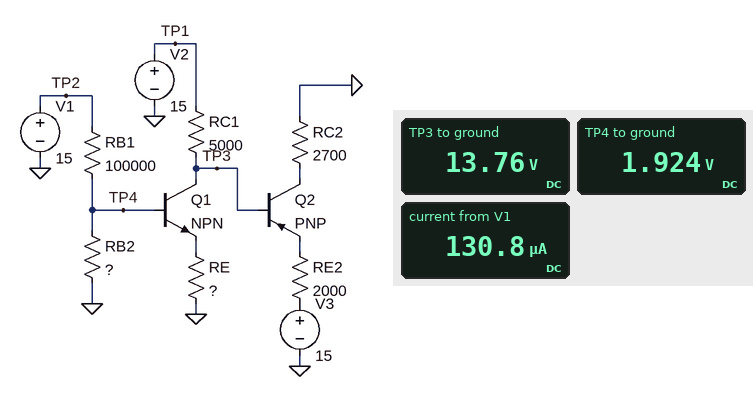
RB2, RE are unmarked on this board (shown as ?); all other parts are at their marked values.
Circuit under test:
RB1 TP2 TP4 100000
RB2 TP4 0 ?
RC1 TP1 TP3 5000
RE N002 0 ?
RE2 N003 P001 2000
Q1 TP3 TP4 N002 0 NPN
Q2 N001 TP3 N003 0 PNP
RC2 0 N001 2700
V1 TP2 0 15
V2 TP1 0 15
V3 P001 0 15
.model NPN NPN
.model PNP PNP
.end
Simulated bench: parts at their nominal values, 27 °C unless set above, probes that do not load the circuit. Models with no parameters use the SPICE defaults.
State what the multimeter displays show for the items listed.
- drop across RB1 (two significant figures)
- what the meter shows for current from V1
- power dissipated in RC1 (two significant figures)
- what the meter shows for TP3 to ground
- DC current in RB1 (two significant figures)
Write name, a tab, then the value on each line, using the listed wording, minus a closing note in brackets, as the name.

drop across RB1	13 V
what the meter shows for current from V1	130.8 µA
power dissipated in RC1	310 µW
what the meter shows for TP3 to ground	13.76 V
DC current in RB1	130 µA
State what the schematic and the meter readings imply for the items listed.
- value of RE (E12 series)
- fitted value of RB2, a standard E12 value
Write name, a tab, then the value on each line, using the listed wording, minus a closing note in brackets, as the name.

value of RE	4.7 kΩ
fitted value of RB2, a standard E12 value	15 kΩ
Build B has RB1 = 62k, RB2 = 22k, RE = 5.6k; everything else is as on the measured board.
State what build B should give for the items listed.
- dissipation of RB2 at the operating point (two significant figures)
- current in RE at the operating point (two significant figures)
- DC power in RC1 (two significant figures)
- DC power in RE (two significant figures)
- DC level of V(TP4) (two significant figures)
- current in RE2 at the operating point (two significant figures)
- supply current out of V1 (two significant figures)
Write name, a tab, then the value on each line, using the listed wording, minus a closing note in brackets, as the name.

dissipation of RB2 at the operating point	670 µW
current in RE at the operating point	550 µA
DC power in RC1	1.4 mW
DC power in RE	1.7 mW
DC level of V(TP4)	3.8 V
current in RE2 at the operating point	950 µA
supply current out of V1	180 µA
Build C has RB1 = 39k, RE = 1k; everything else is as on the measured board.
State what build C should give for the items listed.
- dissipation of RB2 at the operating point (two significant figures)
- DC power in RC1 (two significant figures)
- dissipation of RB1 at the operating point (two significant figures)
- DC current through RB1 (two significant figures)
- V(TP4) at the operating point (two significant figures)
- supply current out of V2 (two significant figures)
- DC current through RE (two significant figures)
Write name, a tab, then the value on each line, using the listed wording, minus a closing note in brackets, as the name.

dissipation of RB2 at the operating point	980 µW
DC power in RC1	15 mW
dissipation of RB1 at the operating point	3.2 mW
DC current through RB1	290 µA
V(TP4) at the operating point	3.8 V
supply current out of V2	1.7 mA
DC current through RE	3.0 mA
